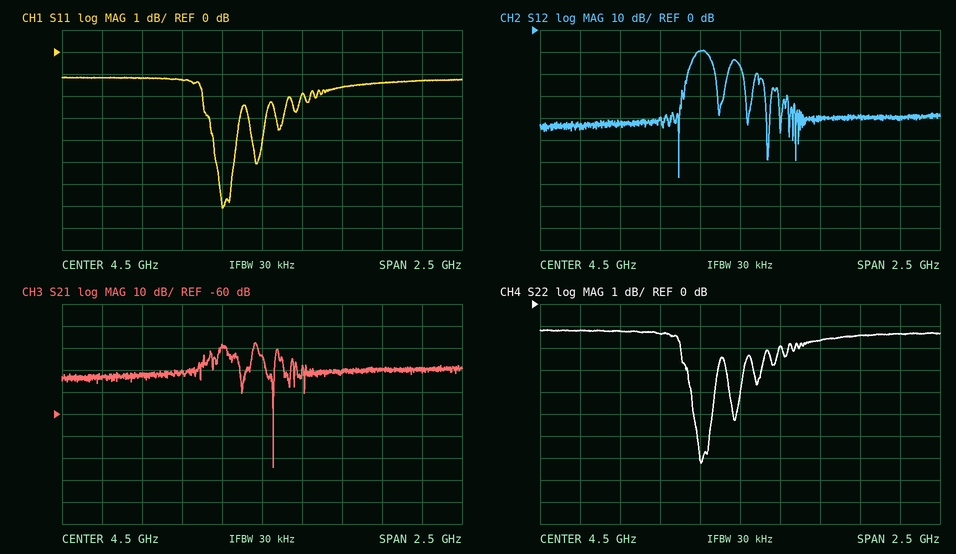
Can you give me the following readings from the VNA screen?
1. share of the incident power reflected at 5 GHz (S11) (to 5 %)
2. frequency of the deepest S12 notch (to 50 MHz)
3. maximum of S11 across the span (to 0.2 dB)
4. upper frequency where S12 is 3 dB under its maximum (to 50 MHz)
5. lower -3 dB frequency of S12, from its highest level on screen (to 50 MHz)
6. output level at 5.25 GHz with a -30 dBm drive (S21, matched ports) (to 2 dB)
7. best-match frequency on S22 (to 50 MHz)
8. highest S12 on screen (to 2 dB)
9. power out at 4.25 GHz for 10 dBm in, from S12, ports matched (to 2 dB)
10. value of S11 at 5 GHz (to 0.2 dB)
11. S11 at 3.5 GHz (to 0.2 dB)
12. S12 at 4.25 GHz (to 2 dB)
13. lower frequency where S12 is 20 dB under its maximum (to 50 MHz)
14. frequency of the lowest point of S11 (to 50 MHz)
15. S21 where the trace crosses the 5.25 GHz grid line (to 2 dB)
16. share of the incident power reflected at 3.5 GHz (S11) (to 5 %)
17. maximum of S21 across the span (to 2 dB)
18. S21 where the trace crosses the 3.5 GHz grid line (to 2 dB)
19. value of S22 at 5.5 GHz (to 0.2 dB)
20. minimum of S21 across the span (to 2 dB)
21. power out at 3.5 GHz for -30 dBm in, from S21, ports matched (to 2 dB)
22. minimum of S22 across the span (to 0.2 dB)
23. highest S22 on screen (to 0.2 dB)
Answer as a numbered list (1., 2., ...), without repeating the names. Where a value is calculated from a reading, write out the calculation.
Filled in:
1. 10^(-1.6/10) ≈ 69.2 %, so 70 % to the nearest 5 %
2. 4.10 GHz
3. -1.2 dB
4. 4.30 GHz
5. 4.20 GHz
6. -30 dBm + (-40 dB) = -70 dBm
7. 4.25 GHz
8. -10 dB
9. 10 dBm + (-10 dB) = 0 dBm
10. -1.6 dB
11. -1.2 dB
12. -10 dB
13. 4.15 GHz
14. 4.25 GHz
15. -40 dB
16. 10^(-1.2/10) ≈ 75.9 %, so 75 % to the nearest 5 %
17. -28 dB
18. -44 dB
19. -1.4 dB
20. -84 dB
21. -30 dBm + (-44 dB) = -74 dBm
22. -7.2 dB
23. -1.2 dB
